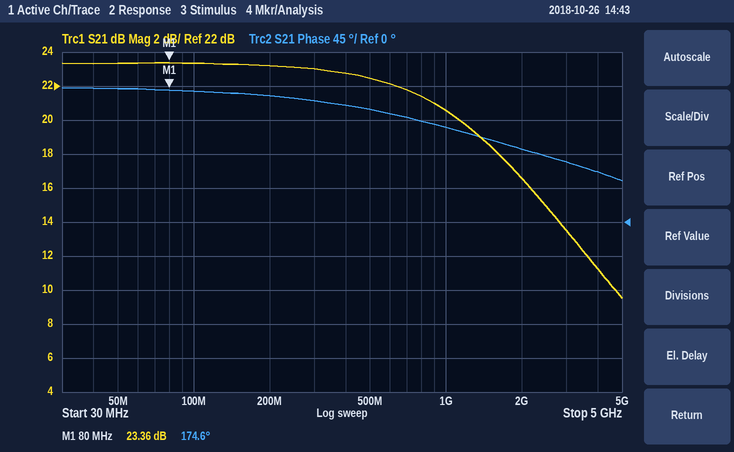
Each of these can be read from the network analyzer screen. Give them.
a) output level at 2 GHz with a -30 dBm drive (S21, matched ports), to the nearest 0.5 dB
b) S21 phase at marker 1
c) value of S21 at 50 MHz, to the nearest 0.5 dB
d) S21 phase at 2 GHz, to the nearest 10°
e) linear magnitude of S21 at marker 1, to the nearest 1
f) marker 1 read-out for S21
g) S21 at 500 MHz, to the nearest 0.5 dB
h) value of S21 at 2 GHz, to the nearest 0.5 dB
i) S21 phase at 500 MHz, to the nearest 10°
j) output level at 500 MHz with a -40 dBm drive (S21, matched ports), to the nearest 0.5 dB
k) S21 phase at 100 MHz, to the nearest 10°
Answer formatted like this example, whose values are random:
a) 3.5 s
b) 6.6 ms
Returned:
a) -13.5 dBm
b) 174.6°
c) 23.5 dB
d) 100°
e) 15
f) 23.36 dB
g) 22.5 dB
h) 16.5 dB
i) 150°
j) -17.5 dBm
k) 170°
